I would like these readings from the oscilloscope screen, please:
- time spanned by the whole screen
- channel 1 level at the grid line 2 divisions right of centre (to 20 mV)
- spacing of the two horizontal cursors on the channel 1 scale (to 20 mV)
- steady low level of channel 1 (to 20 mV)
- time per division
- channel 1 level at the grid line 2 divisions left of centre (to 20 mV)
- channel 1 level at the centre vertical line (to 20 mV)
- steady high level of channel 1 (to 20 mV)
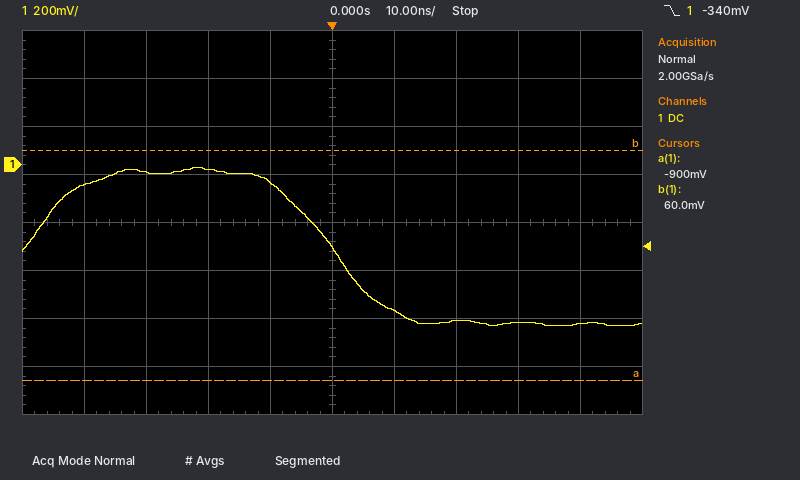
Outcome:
100 ns
-640 mV
960 mV
-660 mV
10 ns
-20 mV
-340 mV
-20 mV
